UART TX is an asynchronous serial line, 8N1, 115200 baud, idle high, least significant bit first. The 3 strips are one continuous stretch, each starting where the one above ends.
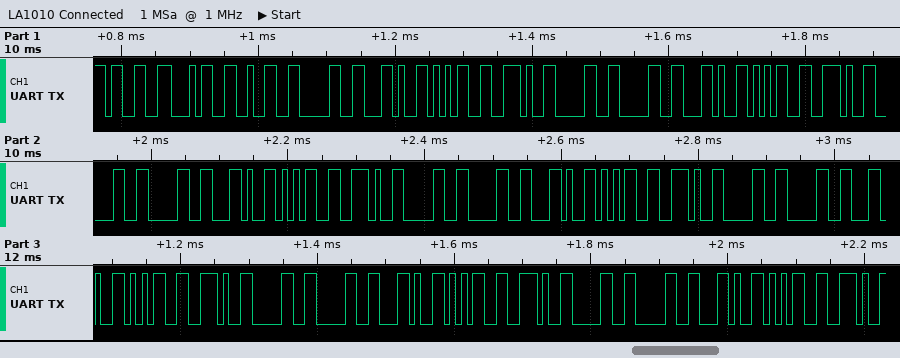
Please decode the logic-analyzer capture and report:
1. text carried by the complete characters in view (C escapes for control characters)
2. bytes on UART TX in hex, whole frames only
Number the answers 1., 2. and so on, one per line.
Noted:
1. "3420,5.00,5.00,5.00,5.00,5.00,5.00,5."
2. 0x33 0x34 0x32 0x30 0x2C 0x35 0x2E 0x30 0x30 0x2C 0x35 0x2E 0x30 0x30 0x2C 0x35 0x2E 0x30 0x30 0x2C 0x35 0x2E 0x30 0x30 0x2C 0x35 0x2E 0x30 0x30 0x2C 0x35 0x2E 0x30 0x30 0x2C 0x35 0x2E
